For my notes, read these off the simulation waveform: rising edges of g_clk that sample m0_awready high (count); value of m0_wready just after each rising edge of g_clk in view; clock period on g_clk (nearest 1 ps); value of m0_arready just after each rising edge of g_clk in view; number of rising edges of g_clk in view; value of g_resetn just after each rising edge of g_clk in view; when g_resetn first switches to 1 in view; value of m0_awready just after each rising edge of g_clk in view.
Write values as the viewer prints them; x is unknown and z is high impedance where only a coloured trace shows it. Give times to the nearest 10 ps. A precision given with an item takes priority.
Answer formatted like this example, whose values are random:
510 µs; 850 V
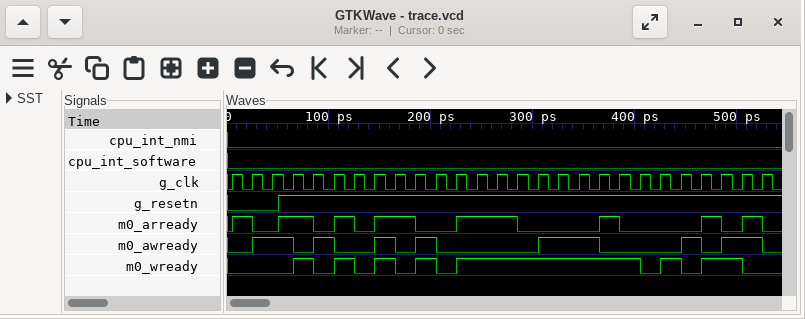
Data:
11; 0 0 0 1 0 1 0 1 0 1 0 1 1 1 1 1 1 1 1 1 0 1 0 1 1 0 0; 20 ps; 1 0 0 1 0 1 0 1 1 0 0 1 1 1 0 0 0 0 1 0 0 0 0 1 0 1 0; 27; 0 0 0 1 1 1 1 1 1 1 1 1 1 1 1 1 1 1 1 1 1 1 1 1 1 1 1; 50 ps; 0 1 1 0 1 0 0 1 0 1 0 0 0 0 0 1 1 1 0 0 0 0 1 0 1 1 0
